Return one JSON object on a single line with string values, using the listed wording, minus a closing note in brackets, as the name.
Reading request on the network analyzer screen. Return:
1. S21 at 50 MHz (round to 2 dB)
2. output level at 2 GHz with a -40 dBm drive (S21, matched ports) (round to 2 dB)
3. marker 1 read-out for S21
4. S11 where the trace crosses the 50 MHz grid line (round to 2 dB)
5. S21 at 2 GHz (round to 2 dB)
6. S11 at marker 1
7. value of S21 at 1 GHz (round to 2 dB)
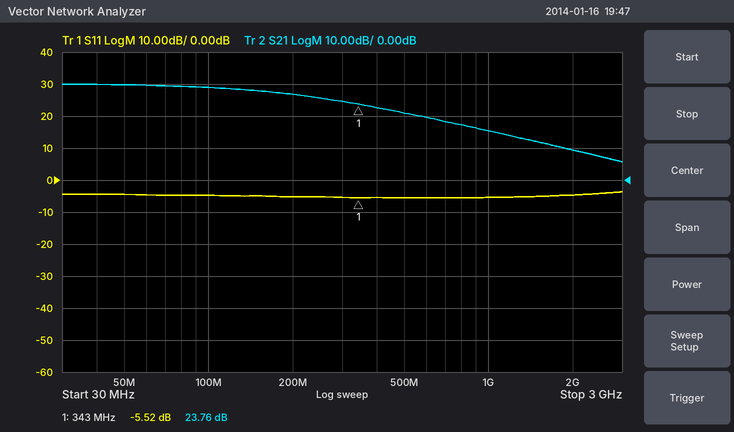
{"S21 at 50 MHz": "30 dB", "output level at 2 GHz with a -40 dBm drive (S21, matched ports)": "-30 dBm", "marker 1 read-out for S21": "23.76 dB", "S11 where the trace crosses the 50 MHz grid line": "-4 dB", "S21 at 2 GHz": "10 dB", "S11 at marker 1": "-5.52 dB", "value of S21 at 1 GHz": "16 dB"}
